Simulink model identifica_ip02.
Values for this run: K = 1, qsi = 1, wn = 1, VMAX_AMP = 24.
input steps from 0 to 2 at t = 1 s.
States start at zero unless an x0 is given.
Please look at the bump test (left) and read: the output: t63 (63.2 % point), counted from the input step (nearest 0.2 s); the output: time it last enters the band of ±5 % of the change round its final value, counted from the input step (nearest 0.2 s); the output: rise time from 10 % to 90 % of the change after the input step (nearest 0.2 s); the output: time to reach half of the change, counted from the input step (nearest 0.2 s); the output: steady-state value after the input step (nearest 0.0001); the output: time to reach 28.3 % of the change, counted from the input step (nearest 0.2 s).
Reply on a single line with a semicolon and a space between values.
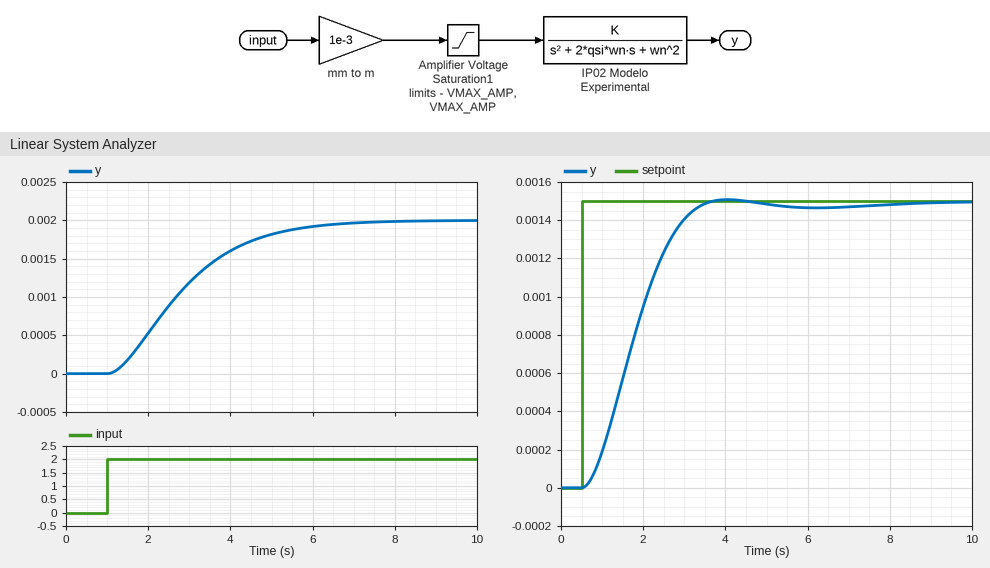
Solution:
2.2 s; 4.8 s; 3.4 s; 1.6 s; 0.0020; 1.0 s
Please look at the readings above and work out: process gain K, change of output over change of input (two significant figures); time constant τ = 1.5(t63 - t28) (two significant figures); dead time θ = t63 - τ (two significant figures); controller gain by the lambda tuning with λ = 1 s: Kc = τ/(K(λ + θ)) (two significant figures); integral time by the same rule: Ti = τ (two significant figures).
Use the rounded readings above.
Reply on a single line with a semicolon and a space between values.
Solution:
0.0010; 1.8 s; 0.40 s; 1300; 1.8 s
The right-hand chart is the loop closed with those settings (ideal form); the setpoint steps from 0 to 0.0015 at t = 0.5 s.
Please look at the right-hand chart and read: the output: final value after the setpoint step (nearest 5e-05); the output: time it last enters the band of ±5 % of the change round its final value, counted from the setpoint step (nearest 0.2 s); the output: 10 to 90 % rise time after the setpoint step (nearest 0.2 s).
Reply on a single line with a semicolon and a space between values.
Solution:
0.00150; 2.6 s; 1.8 s
